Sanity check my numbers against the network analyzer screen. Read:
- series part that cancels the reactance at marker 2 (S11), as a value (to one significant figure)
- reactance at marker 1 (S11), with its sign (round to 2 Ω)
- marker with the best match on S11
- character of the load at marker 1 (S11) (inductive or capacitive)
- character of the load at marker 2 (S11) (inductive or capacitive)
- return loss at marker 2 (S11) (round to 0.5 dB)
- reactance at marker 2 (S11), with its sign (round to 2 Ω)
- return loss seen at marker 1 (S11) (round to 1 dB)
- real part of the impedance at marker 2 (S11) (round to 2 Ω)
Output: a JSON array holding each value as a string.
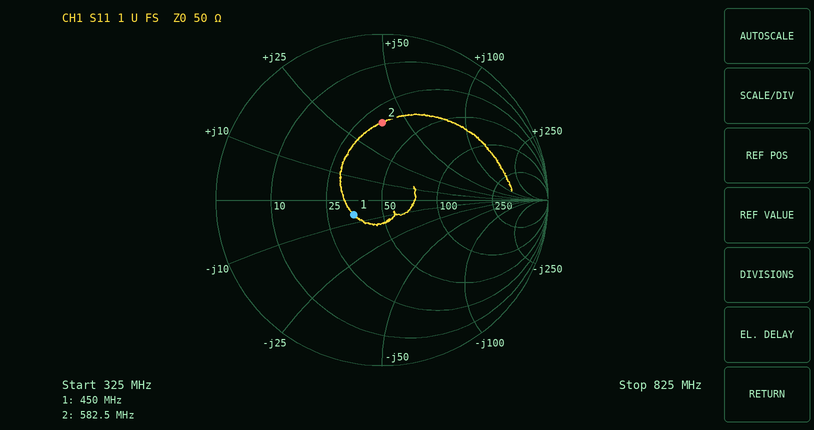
["7 pF", "-6 Ω", "marker 1", "capacitive", "inductive", "6.5 dB", "+38 Ω", "14 dB", "32 Ω"]
